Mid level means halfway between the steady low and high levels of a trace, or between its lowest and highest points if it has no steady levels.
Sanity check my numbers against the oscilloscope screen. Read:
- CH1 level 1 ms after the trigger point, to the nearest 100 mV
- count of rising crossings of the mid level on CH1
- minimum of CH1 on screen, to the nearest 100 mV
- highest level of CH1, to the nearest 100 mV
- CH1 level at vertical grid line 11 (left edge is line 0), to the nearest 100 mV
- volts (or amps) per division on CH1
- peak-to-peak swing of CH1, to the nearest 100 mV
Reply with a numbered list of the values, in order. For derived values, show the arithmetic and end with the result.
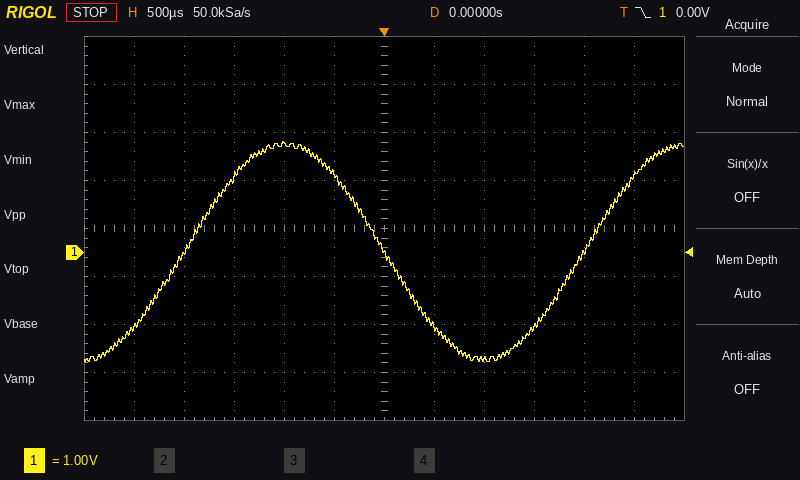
1. -2.2 V
2. 2
3. -2.3 V
4. 2.3 V
5. 1.6 V
6. 1 V
7. 2.3 V − (-2.3 V) = 4.6 V
